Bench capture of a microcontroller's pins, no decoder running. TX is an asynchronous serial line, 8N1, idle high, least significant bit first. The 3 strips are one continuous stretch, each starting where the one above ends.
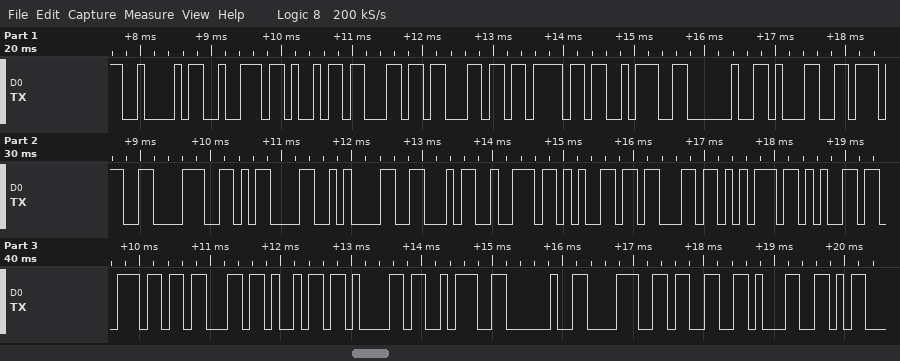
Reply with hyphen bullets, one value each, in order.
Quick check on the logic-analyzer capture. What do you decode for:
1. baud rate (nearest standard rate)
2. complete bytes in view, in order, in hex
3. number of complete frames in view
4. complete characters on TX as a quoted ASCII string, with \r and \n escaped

- 9600 baud
- 42 72 69 6C 6C 6F 3A 20 31 37 38 0D 0A 46 72 65 63 75 65 6E 63 69 61 3A 20 38 33 31
- 28
- "Brillo: 178\r\nFrecuencia: 831"
